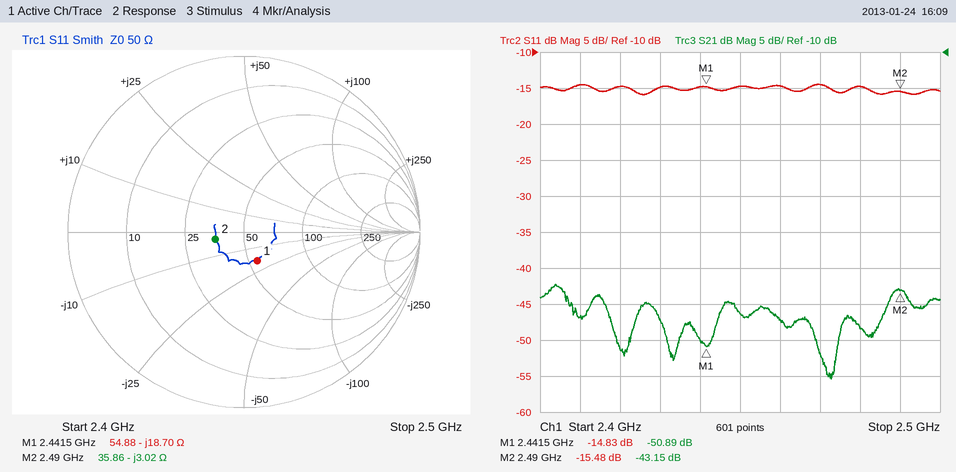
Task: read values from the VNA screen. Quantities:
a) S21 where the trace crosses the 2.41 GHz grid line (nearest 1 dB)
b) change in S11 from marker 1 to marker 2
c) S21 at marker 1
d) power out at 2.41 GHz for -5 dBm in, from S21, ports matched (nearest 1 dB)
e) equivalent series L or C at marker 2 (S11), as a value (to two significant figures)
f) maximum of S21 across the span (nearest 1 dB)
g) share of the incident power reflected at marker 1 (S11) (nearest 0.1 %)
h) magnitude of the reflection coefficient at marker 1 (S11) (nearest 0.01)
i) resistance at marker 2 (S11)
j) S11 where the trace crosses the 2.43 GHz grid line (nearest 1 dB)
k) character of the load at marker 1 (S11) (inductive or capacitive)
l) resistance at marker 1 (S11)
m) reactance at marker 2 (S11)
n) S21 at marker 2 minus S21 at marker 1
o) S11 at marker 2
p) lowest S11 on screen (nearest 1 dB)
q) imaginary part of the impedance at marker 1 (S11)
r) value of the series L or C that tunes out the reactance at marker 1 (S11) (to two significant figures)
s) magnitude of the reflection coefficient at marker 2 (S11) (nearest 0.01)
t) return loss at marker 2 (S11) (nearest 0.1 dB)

-47 dB
-0.65 dB
-50.89 dB
-52 dBm
21 pF
-42 dB
3.3 %
0.18
35.86 Ω
-15 dB
capacitive
54.88 Ω
-3.02 Ω
7.74 dB
-15.48 dB
-16 dB
-18.70 Ω
1.2 nH
0.17
15.5 dB
